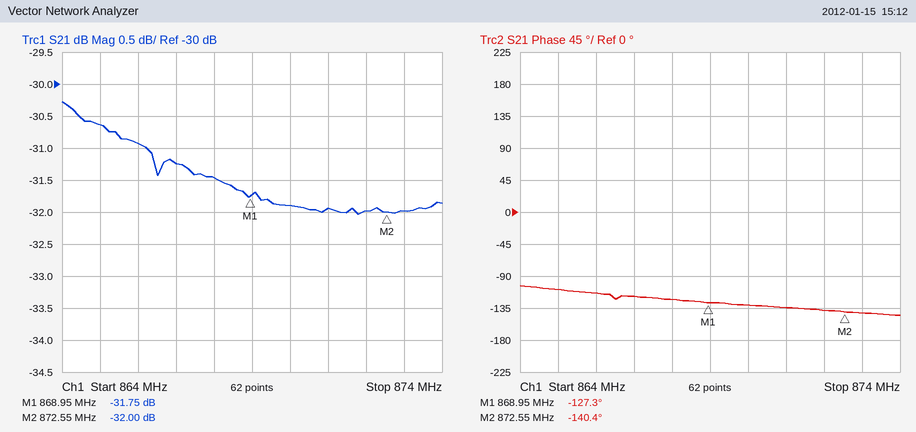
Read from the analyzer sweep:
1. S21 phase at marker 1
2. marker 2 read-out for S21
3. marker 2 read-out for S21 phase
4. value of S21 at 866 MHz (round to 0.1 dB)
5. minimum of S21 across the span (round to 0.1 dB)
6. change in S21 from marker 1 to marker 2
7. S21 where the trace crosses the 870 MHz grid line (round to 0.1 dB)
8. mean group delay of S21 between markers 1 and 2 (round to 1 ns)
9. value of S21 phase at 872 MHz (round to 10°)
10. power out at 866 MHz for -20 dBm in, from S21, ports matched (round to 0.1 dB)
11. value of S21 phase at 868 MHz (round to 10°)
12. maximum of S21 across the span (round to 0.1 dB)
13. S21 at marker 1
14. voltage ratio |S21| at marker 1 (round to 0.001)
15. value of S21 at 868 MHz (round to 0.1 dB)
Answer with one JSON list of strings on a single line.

["-127.3°", "-32.00 dB", "-140.4°", "-30.9 dB", "-32.0 dB", "-0.25 dB", "-31.9 dB", "10 ns", "-140°", "-50.9 dBm", "-120°", "-30.3 dB", "-31.75 dB", "0.026", "-31.5 dB"]
